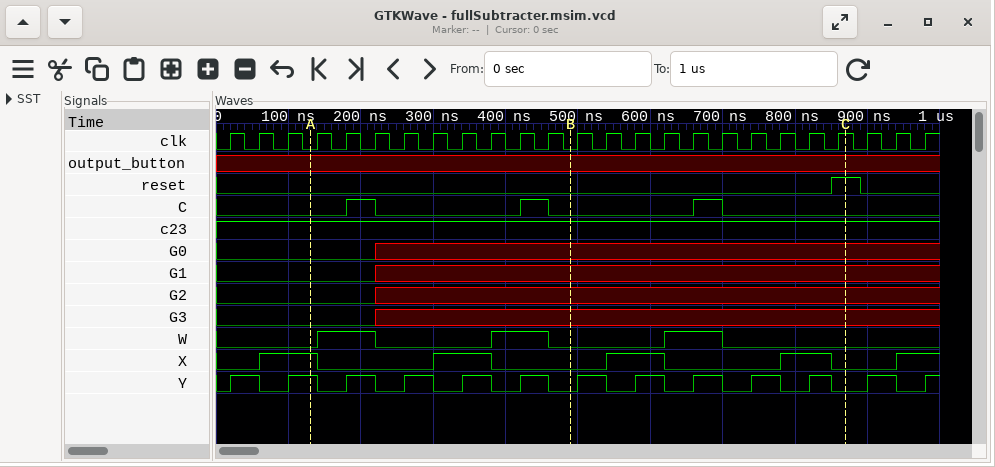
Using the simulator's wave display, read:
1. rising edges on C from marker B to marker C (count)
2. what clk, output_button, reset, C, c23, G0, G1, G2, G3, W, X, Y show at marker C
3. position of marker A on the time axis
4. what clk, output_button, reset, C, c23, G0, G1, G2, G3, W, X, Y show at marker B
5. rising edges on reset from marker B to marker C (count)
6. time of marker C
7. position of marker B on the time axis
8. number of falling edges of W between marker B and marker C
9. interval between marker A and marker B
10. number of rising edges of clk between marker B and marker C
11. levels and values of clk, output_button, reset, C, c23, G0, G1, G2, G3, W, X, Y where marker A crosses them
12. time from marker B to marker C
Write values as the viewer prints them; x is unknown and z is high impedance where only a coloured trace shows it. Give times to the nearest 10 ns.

1
clk=1, output_button=x, reset=1, C=0, c23=1, G0=x, G1=x, G2=x, G3=x, W=0, X=0, Y=0
130 ns
clk=0, output_button=x, reset=0, C=0, c23=1, G0=x, G1=x, G2=x, G3=x, W=0, X=0, Y=0
1
870 ns
490 ns
1
360 ns
10
clk=0, output_button=x, reset=0, C=0, c23=1, G0=0, G1=0, G2=0, G3=0, W=0, X=1, Y=1
380 ns
